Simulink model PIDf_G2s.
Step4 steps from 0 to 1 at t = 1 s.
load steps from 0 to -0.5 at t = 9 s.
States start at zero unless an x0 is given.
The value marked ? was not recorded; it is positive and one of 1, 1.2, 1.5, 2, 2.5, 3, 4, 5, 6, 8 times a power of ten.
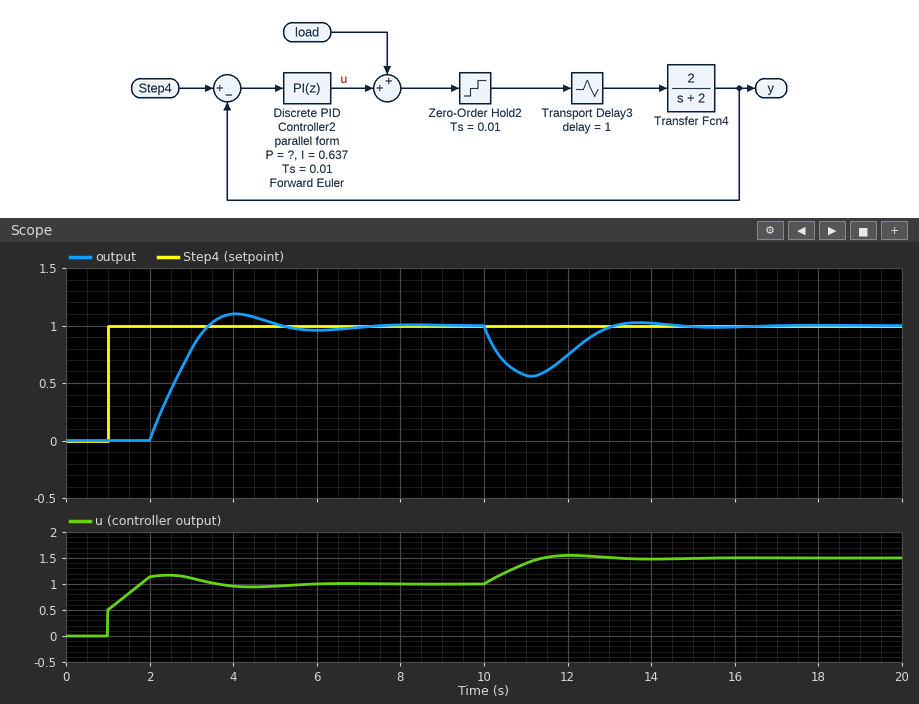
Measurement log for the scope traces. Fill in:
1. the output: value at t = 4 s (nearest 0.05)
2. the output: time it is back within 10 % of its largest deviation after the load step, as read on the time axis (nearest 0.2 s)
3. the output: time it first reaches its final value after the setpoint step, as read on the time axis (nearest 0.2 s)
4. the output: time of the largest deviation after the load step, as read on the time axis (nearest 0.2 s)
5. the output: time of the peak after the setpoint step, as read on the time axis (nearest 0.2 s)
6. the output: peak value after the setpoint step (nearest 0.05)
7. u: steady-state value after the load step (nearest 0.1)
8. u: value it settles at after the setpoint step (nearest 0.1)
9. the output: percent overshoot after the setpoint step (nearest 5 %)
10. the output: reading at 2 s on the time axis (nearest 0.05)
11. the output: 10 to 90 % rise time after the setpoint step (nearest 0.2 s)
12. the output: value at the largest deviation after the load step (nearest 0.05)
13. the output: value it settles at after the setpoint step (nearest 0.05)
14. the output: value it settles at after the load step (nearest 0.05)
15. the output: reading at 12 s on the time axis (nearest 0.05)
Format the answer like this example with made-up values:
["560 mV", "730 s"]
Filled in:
["1.10", "12.8 s", "3.4 s", "11.2 s", "4.0 s", "1.10", "1.5", "1.0", "10 %", "0.00", "1.0 s", "0.55", "1.00", "1.00", "0.75"]
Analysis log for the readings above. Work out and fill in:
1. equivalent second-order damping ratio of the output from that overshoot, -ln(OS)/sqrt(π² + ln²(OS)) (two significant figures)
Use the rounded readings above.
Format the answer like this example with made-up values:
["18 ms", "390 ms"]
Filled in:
["0.59"]
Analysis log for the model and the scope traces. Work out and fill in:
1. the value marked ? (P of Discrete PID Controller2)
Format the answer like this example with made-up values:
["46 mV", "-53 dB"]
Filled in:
["0.5"]
